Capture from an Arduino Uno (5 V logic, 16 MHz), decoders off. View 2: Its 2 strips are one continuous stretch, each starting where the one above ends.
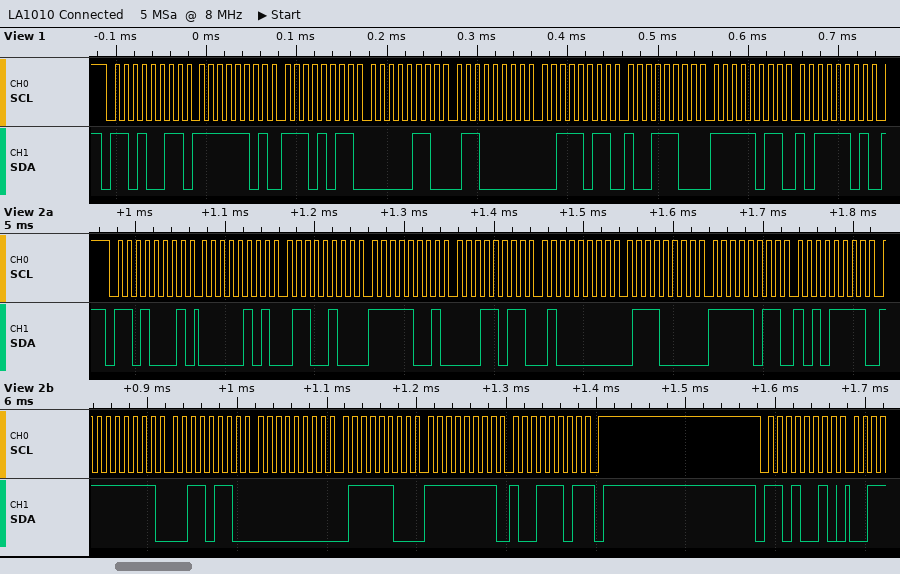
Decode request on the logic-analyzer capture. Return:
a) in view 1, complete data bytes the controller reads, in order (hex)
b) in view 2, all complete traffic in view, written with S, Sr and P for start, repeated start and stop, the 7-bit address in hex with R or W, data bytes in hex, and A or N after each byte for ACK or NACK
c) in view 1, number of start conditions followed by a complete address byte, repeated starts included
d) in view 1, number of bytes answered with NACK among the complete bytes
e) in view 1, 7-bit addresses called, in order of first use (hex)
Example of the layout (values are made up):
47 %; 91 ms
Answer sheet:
FD EB 06 60 3B 9C FB BD; S 68R A 05 A 64 A F9 A 1B A 40 A 70 A FB A AF A FF A 36 A 00 A 7C A FF A 9D N P S 69W A; 1; 0; 0x69
